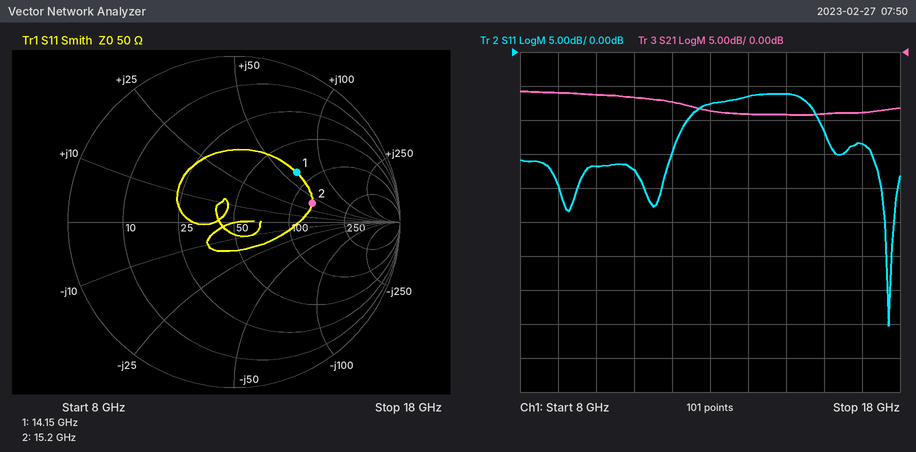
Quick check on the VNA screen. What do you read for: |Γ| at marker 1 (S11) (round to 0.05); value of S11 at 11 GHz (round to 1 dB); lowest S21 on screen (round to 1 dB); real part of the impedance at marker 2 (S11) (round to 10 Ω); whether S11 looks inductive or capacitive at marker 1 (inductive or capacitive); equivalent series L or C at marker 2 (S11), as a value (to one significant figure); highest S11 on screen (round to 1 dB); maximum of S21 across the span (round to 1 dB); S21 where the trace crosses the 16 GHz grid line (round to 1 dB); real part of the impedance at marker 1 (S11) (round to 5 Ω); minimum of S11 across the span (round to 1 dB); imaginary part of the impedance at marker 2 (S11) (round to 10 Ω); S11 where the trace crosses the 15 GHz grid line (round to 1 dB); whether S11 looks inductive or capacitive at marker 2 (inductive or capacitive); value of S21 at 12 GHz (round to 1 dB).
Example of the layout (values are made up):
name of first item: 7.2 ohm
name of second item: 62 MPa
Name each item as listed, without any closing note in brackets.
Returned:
|Γ| at marker 1 (S11): 0.50
value of S11 at 11 GHz: -17 dB
lowest S21 on screen: -9 dB
real part of the impedance at marker 2 (S11): 130 Ω
whether S11 looks inductive or capacitive at marker 1: inductive
equivalent series L or C at marker 2 (S11), as a value: 400 pH
highest S11 on screen: -6 dB
maximum of S21 across the span: -6 dB
S21 where the trace crosses the 16 GHz grid line: -9 dB
real part of the impedance at marker 1 (S11): 80 Ω
minimum of S11 across the span: -40 dB
imaginary part of the impedance at marker 2 (S11): +40 Ω
S11 where the trace crosses the 15 GHz grid line: -6 dB
whether S11 looks inductive or capacitive at marker 2: inductive
value of S21 at 12 GHz: -7 dB
